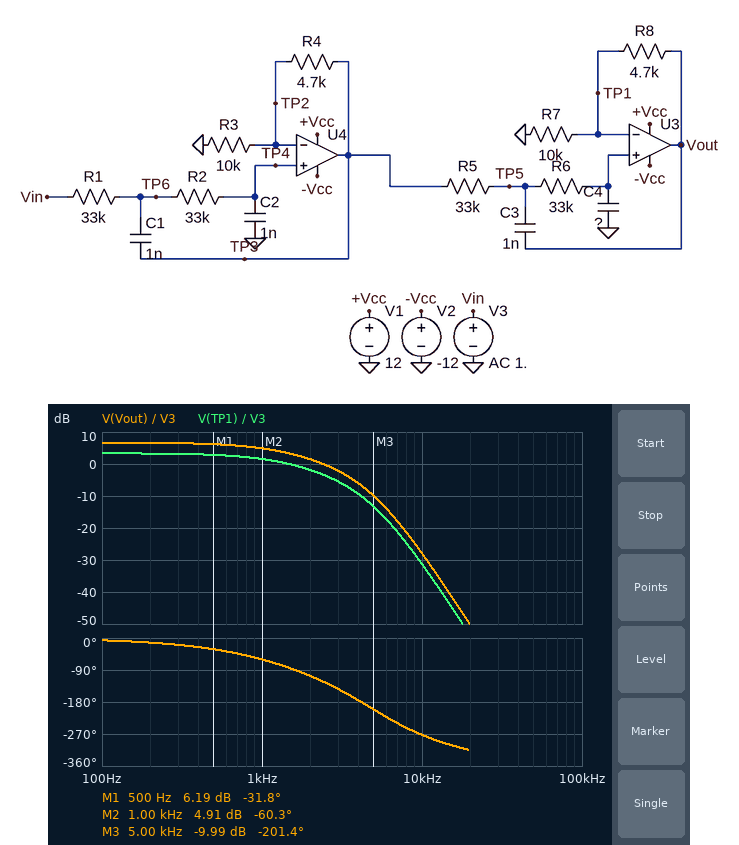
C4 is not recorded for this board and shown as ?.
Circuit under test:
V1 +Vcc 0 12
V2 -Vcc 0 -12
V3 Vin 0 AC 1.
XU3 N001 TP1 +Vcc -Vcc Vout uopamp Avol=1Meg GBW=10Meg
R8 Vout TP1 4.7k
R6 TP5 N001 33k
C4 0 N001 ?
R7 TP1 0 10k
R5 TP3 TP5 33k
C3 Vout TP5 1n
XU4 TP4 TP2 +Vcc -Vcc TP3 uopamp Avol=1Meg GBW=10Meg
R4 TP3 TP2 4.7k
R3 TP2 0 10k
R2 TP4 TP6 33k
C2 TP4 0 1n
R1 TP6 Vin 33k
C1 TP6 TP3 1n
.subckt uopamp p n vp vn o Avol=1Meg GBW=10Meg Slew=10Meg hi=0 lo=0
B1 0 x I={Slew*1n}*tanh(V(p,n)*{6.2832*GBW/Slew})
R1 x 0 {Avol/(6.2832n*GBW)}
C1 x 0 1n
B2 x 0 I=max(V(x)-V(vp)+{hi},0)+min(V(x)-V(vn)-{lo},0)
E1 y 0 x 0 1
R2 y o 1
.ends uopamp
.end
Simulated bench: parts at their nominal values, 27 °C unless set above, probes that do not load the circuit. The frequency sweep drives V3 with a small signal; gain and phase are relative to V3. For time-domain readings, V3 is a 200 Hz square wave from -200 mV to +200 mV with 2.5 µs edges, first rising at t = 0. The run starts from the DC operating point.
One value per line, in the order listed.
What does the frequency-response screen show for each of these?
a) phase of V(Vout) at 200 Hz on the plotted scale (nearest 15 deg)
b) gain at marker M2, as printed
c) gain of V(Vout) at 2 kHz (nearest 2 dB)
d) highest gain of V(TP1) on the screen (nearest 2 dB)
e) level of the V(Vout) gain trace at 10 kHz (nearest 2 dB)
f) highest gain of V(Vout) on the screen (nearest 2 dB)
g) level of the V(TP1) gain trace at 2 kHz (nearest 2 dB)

-15 deg
4.91 dB
2 dB
4 dB
-28 dB
6 dB
-2 dB
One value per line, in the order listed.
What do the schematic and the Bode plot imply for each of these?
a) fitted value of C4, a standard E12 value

2.2 nF
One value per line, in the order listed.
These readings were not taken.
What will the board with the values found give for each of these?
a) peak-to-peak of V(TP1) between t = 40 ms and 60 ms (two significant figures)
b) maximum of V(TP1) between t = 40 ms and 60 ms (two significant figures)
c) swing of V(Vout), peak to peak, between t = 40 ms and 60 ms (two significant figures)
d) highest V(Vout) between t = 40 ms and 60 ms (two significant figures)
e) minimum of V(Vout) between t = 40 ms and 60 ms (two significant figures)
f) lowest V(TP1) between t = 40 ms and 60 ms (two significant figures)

590 mV
290 mV
860 mV
430 mV
-430 mV
-290 mV
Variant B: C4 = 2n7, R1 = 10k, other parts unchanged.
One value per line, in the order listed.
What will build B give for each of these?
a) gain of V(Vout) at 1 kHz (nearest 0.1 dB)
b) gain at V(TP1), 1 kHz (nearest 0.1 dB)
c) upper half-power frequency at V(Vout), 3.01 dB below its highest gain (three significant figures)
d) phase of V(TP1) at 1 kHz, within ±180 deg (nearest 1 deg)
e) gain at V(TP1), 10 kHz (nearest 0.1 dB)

3.9 dB
0.6 dB
1.06 kHz
-63 deg
-27.7 dB
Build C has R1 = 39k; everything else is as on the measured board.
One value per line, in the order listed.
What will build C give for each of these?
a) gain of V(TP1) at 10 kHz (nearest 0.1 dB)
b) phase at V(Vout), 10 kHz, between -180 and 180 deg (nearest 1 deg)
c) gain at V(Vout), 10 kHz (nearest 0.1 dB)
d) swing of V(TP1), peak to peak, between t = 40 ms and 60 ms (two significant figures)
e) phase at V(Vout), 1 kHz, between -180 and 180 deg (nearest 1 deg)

-32.5 dB
83 deg
-29.2 dB
590 mV
-62 deg
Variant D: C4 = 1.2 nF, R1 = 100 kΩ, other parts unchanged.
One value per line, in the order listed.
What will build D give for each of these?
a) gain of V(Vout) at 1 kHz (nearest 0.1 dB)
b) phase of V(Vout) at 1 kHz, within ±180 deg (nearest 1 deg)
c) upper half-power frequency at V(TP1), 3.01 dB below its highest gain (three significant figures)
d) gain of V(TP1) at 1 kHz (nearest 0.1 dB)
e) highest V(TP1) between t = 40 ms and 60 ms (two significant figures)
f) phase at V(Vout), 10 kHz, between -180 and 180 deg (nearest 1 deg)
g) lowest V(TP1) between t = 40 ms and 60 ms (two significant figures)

6.2 dB
-55 deg
2.16 kHz
2.9 dB
310 mV
68 deg
-310 mV
